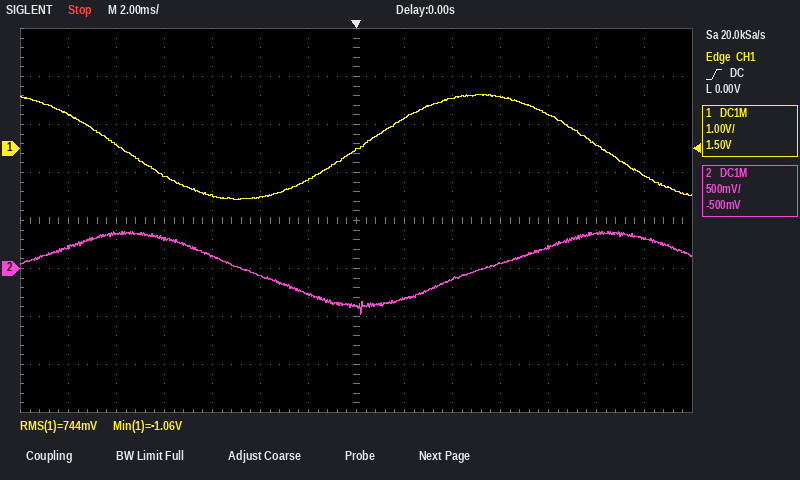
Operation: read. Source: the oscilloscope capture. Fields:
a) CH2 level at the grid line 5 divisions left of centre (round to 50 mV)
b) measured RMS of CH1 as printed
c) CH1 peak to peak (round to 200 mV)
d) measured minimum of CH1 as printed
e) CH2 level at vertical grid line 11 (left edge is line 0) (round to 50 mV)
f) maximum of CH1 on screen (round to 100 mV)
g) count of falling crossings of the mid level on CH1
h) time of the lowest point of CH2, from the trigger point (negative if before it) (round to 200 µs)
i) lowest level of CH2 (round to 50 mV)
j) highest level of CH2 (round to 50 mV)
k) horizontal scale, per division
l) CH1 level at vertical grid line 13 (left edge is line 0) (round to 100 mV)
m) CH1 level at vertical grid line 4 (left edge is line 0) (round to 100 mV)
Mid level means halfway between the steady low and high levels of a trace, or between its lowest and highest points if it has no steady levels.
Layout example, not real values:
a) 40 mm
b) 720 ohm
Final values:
a) 350 mV
b) 744 mV
c) 2.2 V
d) -1.06 V
e) 200 mV
f) 1.1 V
g) 2
h) +200 µs
i) -500 mV
j) 400 mV
k) 2 ms
l) -600 mV
m) -1.0 V
